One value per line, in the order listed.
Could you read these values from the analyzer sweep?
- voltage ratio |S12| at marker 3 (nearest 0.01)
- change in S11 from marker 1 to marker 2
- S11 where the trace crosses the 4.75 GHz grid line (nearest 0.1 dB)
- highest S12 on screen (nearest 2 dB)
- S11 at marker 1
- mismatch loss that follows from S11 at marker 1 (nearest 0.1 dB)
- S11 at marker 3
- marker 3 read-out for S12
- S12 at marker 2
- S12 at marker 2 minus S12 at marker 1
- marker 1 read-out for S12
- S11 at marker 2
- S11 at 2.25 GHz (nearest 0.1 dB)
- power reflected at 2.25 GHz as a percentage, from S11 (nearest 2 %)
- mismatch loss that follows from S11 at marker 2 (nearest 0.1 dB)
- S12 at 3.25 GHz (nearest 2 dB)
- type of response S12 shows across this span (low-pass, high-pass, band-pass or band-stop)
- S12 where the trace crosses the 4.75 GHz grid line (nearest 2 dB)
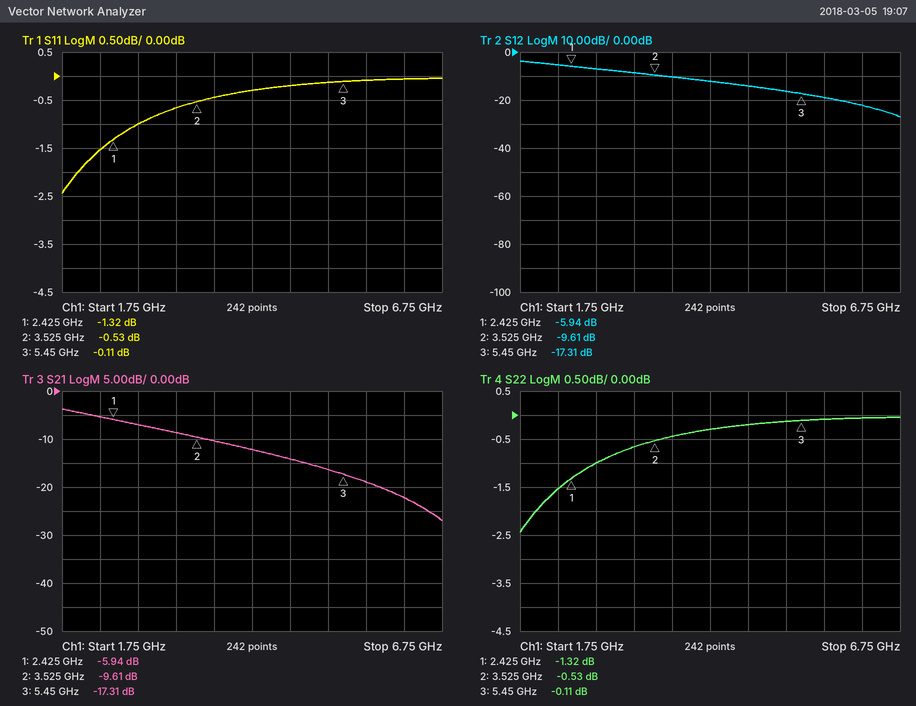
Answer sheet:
0.14
0.79 dB
-0.2 dB
-4 dB
-1.32 dB
5.8 dB
-0.11 dB
-17.31 dB
-9.61 dB
-3.67 dB
-5.94 dB
-0.53 dB
-1.5 dB
70 %
9.4 dB
-8 dB
low-pass
-14 dB
